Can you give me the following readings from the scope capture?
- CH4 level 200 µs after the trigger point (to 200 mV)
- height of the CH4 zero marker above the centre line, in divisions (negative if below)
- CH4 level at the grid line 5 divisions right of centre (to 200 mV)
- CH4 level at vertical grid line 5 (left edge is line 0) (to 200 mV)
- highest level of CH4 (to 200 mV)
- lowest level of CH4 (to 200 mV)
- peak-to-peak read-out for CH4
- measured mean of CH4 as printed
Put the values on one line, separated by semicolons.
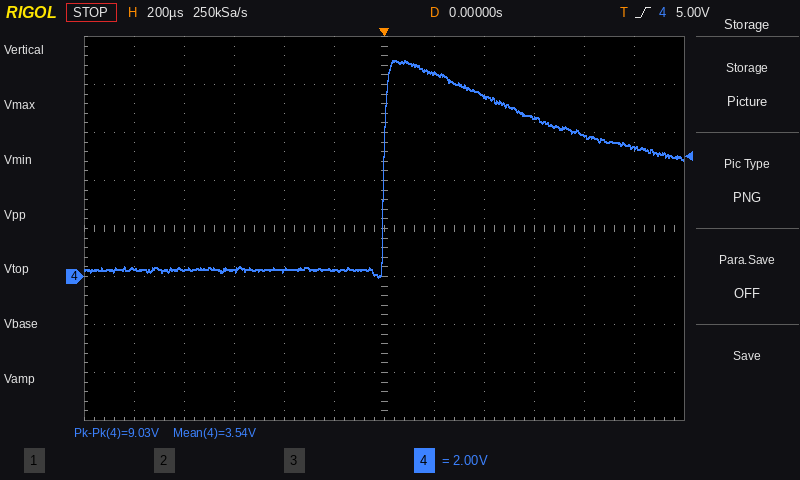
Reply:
8.4 V; -1.0 div; 5.4 V; 200 mV; 9.0 V; 0.0 V; 9.03 V; 3.54 V
